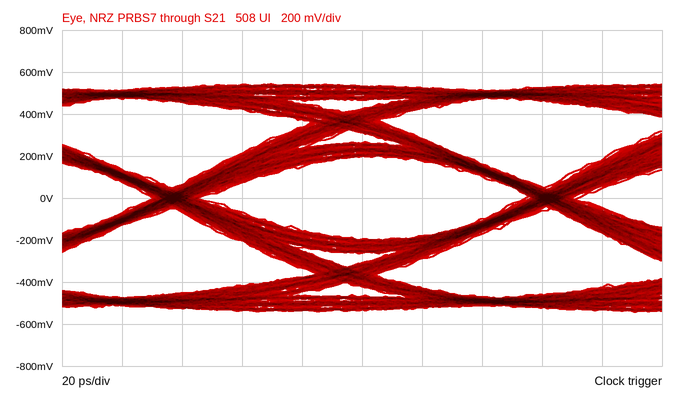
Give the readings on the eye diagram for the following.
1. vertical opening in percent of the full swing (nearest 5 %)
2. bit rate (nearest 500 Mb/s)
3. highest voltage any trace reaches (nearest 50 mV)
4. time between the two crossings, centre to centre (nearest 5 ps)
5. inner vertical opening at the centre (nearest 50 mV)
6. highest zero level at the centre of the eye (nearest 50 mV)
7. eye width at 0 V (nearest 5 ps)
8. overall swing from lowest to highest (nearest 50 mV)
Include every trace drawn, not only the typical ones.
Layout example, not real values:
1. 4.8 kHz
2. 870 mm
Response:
1. 35 %
2. 8.0 Gb/s
3. 550 mV
4. 125 ps
5. 400 mV
6. -200 mV
7. 110 ps
8. 1.10 V
